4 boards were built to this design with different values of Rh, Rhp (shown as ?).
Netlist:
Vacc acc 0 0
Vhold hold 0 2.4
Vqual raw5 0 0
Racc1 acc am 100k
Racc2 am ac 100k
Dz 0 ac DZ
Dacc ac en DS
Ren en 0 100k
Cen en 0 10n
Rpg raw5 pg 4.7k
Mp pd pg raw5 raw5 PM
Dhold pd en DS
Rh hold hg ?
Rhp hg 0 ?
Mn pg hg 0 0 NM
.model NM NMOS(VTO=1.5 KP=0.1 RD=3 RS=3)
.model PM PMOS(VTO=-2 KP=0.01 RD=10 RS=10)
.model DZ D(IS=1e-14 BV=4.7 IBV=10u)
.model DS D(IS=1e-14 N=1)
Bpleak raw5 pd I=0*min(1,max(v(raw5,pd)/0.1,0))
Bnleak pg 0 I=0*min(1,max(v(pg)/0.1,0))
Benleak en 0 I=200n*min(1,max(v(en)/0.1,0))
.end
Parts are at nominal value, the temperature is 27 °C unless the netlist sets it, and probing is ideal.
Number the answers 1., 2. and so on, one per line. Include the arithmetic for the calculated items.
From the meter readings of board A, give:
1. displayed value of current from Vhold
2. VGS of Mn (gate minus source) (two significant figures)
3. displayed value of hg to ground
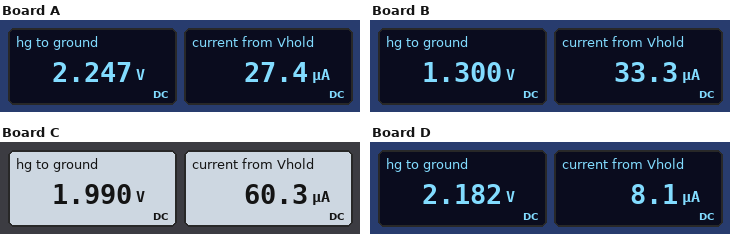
1. 27.4 µA
2. 2.247 V = 2.2 V
3. 2.247 V
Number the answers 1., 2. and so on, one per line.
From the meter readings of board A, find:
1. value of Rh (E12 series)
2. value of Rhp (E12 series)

1. 5.6 kΩ
2. 82 kΩ
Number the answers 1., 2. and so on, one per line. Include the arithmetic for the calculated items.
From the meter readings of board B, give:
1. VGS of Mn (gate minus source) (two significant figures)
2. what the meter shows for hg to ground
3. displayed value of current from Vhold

1. 1.3 V = 1.3 V
2. 1.300 V
3. 33.3 µA
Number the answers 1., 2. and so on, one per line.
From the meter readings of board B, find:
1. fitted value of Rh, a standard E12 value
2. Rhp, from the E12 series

1. 33 kΩ
2. 39 kΩ
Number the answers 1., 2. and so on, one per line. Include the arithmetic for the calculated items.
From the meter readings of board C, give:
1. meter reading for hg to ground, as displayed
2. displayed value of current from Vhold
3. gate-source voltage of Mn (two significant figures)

1. 1.990 V
2. 60.3 µA
3. 1.99 V = 2.0 V
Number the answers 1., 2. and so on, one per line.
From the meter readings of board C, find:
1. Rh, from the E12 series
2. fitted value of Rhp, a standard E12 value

1. 6.8 kΩ
2. 33 kΩ
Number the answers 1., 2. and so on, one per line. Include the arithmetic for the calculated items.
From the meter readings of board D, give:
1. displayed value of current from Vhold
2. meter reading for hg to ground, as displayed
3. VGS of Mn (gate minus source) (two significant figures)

1. 8.1 µA
2. 2.182 V
3. 2.182 V = 2.2 V
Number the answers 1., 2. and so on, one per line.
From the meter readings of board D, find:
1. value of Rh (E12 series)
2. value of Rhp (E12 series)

1. 27 kΩ
2. 270 kΩ
